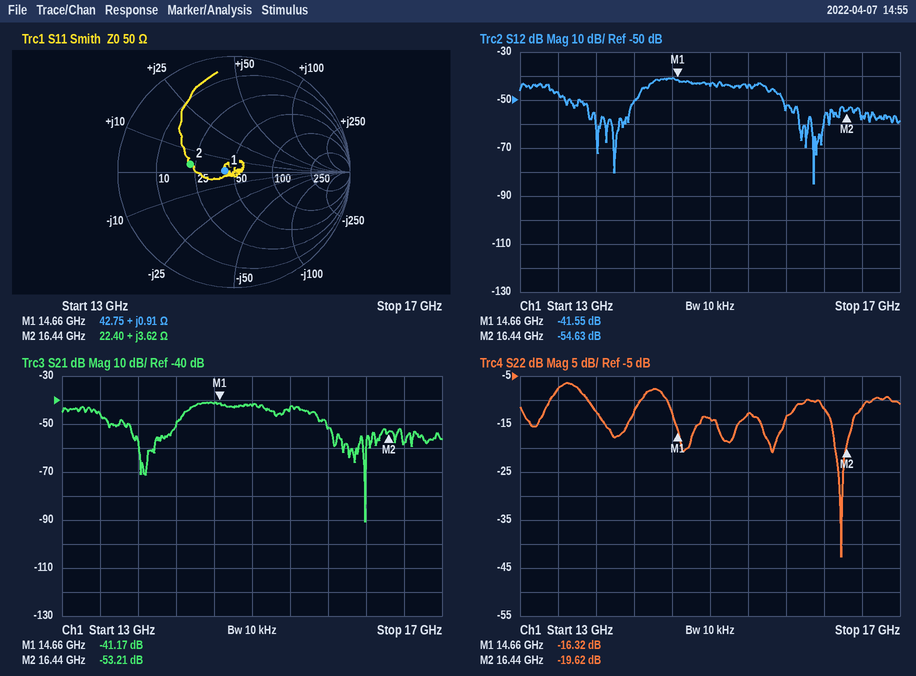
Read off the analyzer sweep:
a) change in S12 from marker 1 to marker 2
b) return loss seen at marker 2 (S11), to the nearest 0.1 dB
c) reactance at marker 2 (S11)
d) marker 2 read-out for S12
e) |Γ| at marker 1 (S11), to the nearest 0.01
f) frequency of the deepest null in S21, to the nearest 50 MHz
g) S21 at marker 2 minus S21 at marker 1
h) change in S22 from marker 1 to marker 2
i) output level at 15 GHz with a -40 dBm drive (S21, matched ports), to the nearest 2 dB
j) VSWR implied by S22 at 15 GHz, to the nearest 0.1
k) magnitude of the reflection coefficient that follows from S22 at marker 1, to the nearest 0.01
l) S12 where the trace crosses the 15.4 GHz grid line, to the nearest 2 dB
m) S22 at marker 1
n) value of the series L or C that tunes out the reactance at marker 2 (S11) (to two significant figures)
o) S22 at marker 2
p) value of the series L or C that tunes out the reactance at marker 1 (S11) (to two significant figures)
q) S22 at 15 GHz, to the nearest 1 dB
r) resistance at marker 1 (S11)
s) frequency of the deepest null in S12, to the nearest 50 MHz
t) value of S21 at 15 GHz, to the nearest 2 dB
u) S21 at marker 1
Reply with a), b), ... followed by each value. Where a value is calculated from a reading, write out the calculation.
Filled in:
a) -54.63 − (-41.55) = -13.08 dB
b) 8.3 dB
c) +3.62 Ω
d) -54.63 dB
e) 0.08
f) 16.20 GHz
g) -53.21 − (-41.17) = -12.04 dB
h) -19.62 − (-16.32) = -3.30 dB
i) -40 dBm + (-42 dB) = -82 dBm
j) |Γ| = 10^(-14/20) = 0.1995; VSWR = (1 + 0.1995)/(1 − 0.1995) ≈ 1.5
k) 10^(-16.32/20) ≈ 0.15
l) -44 dB
m) -16.32 dB
n) C = 1/(2π × 16.44 GHz × 3.62 Ω) ≈ 2.7 pF
o) -19.62 dB
p) C = 1/(2π × 14.66 GHz × 0.91 Ω) ≈ 12 pF
q) -14 dB
r) 42.75 Ω
s) 16.10 GHz
t) -42 dB
u) -41.17 dB
